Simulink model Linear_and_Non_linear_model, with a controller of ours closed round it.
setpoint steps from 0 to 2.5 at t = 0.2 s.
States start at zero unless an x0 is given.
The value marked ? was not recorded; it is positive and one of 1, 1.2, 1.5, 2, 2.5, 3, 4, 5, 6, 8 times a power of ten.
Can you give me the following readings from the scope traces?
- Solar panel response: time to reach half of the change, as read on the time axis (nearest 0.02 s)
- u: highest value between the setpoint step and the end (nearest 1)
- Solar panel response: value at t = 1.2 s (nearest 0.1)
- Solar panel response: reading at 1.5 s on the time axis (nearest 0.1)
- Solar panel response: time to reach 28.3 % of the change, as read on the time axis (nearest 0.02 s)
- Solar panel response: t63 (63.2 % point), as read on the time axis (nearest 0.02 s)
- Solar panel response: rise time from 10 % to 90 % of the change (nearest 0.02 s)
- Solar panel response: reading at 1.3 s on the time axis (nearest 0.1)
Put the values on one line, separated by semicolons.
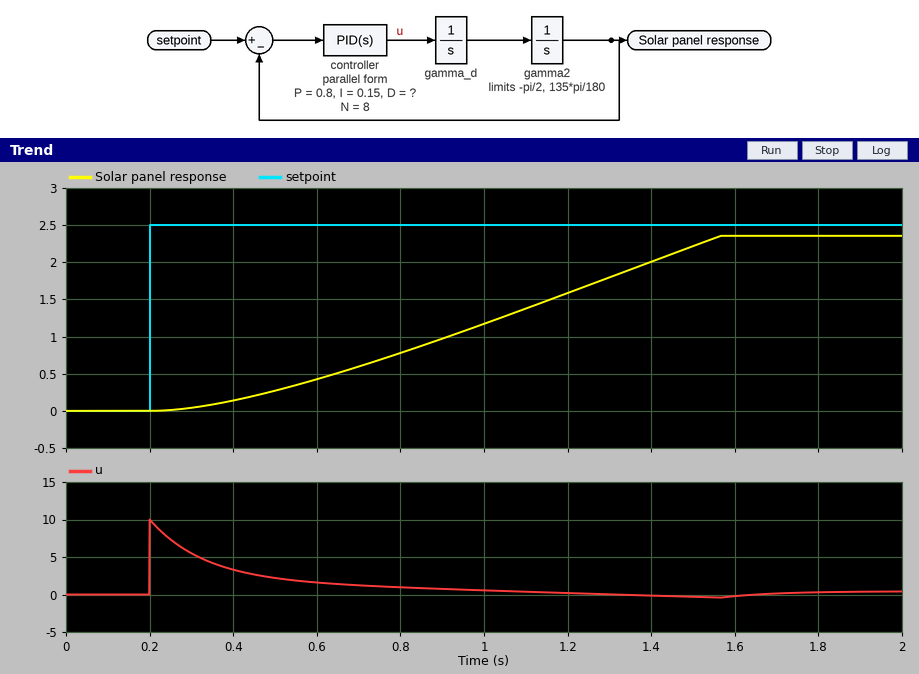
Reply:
1.00 s; 10; 1.6; 2.2; 0.74 s; 1.16 s; 0.98 s; 1.8
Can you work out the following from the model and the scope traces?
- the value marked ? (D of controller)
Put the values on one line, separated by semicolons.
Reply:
0.4
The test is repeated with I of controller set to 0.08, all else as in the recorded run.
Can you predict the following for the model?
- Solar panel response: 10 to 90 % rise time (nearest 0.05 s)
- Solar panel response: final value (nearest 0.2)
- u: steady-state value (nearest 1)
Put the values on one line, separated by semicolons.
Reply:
1.00 s; 2.4; 0
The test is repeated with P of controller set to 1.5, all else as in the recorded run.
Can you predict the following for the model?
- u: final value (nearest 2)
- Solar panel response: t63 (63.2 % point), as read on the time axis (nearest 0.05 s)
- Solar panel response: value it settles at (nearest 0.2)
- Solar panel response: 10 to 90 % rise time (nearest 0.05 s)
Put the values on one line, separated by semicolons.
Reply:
0; 0.95 s; 2.4; 0.75 s
